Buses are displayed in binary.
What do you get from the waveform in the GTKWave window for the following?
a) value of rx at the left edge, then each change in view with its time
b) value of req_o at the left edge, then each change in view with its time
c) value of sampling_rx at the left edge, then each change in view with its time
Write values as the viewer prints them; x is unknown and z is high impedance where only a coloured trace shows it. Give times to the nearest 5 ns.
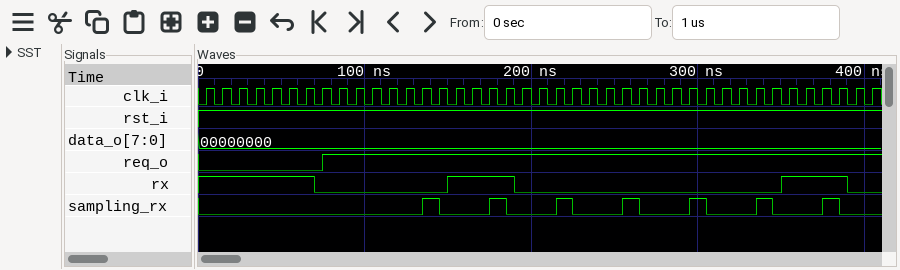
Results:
1, 0 at 70 ns, 1 at 150 ns, 0 at 190 ns, 1 at 350 ns, 0 at 390 ns
0, 1 at 75 ns
0, 1 at 135 ns, 0 at 145 ns, 1 at 175 ns, 0 at 185 ns, 1 at 215 ns, 0 at 225 ns, 1 at 255 ns, 0 at 265 ns, 1 at 295 ns, 0 at 305 ns, 1 at 335 ns, 0 at 345 ns, 1 at 375 ns, 0 at 385 ns
